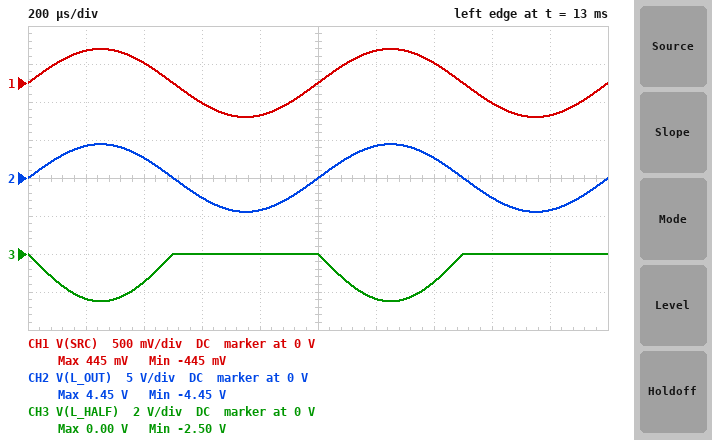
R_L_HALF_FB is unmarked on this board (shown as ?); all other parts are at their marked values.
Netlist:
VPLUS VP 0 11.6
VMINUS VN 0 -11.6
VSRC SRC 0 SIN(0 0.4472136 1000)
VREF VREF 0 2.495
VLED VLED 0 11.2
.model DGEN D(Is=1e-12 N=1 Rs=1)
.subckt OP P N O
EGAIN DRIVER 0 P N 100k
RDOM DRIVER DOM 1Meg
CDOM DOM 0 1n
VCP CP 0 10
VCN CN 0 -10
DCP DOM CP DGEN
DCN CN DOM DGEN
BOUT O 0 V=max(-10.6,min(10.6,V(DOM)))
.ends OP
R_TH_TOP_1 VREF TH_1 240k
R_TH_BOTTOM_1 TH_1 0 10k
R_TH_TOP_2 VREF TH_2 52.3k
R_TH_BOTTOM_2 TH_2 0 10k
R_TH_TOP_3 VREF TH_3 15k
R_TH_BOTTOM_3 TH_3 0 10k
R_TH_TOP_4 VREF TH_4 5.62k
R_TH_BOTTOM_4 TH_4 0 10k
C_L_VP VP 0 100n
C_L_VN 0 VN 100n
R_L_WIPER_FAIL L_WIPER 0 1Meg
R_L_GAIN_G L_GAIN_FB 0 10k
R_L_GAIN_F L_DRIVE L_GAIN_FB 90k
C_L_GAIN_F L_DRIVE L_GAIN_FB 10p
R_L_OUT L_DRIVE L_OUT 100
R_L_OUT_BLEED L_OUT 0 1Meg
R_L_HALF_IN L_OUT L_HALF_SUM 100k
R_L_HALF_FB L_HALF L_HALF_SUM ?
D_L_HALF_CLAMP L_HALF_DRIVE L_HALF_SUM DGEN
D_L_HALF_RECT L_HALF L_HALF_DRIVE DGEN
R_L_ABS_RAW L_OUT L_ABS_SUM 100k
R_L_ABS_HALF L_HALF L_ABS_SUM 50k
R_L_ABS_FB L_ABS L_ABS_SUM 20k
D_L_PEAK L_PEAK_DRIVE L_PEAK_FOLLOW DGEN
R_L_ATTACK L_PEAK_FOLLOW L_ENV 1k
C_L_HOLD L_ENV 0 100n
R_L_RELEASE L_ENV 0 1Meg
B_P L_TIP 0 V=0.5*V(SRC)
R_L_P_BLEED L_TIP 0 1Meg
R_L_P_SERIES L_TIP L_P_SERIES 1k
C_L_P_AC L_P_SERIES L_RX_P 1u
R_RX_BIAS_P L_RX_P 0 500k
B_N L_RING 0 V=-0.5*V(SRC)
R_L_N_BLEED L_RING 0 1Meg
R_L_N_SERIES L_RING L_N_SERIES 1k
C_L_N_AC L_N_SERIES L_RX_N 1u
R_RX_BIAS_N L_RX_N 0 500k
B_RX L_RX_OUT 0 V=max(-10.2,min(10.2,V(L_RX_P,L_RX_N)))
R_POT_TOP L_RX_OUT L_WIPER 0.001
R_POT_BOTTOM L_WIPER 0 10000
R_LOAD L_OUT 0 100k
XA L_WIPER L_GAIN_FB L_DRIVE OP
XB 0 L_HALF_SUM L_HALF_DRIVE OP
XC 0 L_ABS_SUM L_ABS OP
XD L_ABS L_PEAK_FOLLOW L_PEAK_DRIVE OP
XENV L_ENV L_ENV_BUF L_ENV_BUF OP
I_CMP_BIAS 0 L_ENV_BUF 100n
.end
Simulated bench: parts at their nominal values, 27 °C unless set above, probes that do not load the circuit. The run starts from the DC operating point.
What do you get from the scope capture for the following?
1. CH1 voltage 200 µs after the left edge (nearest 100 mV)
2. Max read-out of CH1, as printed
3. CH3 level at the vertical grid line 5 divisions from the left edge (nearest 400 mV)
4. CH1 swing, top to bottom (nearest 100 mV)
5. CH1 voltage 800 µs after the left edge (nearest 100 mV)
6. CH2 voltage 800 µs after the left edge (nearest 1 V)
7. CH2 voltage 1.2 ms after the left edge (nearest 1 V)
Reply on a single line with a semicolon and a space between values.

400 mV; 445 mV; 0 V; 900 mV; -400 mV; -4 V; 4 V
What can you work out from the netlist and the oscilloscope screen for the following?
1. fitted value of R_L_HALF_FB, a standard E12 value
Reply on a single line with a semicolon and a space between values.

56 kΩ
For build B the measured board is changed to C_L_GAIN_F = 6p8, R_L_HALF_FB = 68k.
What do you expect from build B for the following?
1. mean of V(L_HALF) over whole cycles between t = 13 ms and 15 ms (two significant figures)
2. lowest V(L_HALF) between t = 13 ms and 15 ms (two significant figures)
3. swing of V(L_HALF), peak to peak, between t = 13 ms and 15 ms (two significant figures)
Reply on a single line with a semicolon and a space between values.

-960 mV; -3.0 V; 3.0 V
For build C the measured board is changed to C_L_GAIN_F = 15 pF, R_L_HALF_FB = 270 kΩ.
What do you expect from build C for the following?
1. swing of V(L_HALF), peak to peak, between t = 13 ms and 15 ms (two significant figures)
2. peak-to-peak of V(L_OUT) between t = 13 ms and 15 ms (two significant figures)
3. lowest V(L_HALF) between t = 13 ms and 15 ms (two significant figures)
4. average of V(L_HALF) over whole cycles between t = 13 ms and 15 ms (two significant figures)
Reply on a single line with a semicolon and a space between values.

10 V; 8.9 V; -10 V; -3.6 V
